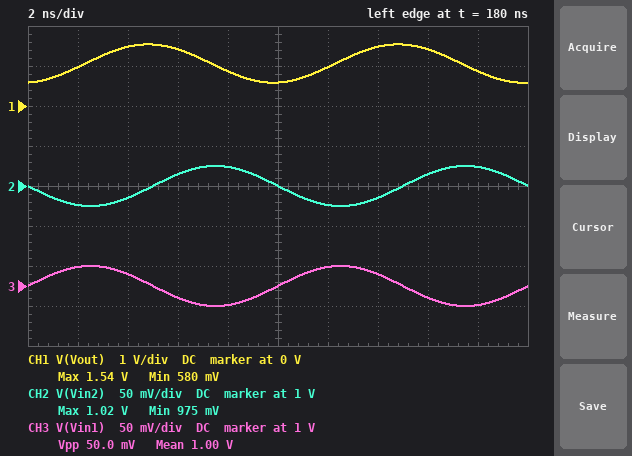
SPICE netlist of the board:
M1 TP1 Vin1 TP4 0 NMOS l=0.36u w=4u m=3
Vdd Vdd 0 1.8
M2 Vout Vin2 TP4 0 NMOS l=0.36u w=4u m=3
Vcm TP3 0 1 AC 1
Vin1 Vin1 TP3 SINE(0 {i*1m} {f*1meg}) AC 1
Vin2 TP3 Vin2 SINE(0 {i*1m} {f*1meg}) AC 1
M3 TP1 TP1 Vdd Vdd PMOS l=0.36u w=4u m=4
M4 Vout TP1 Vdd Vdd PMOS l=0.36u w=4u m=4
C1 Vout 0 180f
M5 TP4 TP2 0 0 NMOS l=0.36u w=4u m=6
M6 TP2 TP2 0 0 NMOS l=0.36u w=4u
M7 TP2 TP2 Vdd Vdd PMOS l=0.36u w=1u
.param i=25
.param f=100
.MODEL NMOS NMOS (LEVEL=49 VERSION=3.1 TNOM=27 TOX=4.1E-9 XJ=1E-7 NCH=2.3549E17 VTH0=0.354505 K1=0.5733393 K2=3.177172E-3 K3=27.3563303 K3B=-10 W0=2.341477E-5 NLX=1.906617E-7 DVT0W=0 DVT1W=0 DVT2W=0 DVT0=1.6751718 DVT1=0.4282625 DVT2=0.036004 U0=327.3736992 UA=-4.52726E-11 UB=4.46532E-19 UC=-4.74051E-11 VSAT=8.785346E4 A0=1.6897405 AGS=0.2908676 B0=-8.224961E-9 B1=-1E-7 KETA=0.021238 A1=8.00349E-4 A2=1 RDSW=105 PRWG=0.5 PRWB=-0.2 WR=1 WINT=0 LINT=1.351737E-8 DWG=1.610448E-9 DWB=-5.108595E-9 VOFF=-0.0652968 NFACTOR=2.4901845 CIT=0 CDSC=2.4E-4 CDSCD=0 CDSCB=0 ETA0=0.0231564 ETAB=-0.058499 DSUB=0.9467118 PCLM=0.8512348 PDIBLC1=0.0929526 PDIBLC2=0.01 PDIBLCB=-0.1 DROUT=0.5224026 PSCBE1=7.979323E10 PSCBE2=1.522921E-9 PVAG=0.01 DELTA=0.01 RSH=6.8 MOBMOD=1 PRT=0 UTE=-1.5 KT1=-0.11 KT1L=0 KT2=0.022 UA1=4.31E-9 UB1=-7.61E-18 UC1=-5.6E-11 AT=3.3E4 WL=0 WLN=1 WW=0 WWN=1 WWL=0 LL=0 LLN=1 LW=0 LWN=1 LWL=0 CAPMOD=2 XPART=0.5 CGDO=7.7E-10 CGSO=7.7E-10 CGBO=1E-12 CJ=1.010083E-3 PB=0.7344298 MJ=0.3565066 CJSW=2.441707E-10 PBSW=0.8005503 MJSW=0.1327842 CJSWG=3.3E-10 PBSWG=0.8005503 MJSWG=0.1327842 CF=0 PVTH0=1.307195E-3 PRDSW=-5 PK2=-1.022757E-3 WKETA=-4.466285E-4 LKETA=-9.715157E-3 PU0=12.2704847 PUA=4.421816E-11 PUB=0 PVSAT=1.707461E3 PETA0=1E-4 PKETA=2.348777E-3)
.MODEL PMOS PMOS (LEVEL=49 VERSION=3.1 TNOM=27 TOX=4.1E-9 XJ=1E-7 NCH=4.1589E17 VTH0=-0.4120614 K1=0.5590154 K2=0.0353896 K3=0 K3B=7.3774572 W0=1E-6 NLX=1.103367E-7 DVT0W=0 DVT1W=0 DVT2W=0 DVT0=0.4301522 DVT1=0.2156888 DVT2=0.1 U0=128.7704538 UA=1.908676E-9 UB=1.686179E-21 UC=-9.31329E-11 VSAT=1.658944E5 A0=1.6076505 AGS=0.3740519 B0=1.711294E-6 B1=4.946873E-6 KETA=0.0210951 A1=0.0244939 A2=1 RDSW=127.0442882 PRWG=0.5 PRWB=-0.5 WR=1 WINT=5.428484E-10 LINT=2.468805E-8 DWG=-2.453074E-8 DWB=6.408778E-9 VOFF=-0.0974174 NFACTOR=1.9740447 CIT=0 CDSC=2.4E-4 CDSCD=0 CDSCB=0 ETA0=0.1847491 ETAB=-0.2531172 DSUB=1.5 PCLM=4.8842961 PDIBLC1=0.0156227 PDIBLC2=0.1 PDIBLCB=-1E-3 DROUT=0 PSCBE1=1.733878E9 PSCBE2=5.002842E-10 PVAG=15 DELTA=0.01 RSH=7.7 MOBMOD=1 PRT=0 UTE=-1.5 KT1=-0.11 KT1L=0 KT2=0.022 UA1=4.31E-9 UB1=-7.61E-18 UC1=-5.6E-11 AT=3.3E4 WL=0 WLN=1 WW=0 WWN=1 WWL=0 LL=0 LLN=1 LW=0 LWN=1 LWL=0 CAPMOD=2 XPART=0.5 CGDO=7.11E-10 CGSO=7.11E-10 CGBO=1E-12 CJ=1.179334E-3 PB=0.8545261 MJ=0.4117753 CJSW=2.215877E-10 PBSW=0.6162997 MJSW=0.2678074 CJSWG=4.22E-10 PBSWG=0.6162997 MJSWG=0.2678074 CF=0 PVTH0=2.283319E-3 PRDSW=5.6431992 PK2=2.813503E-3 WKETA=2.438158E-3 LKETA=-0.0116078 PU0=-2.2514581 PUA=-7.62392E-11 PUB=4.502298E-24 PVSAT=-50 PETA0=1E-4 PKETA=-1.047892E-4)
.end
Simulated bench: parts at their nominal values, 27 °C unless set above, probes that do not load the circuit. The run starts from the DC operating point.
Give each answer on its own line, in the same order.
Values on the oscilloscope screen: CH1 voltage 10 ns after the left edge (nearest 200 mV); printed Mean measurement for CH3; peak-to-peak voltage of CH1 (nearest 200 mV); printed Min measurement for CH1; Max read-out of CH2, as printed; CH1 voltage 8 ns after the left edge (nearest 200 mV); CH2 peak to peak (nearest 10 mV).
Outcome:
600 mV
1.00 V
1.0 V
580 mV
1.02 V
800 mV
50 mV
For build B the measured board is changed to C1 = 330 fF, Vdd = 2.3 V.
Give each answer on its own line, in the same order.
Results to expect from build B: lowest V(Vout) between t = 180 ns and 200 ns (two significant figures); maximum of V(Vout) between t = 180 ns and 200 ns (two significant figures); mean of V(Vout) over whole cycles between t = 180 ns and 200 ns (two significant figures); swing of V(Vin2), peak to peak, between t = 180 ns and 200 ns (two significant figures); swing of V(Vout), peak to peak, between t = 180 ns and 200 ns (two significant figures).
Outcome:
1.0 V
1.8 V
1.4 V
50 mV
830 mV
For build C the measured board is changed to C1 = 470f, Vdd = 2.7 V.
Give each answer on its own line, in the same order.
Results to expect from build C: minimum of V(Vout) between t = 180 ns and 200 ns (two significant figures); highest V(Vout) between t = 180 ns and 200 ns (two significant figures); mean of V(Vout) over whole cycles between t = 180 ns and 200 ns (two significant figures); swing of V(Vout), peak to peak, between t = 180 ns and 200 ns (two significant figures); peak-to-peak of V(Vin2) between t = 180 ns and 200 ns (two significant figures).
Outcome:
1.4 V
2.1 V
1.7 V
680 mV
50 mV
